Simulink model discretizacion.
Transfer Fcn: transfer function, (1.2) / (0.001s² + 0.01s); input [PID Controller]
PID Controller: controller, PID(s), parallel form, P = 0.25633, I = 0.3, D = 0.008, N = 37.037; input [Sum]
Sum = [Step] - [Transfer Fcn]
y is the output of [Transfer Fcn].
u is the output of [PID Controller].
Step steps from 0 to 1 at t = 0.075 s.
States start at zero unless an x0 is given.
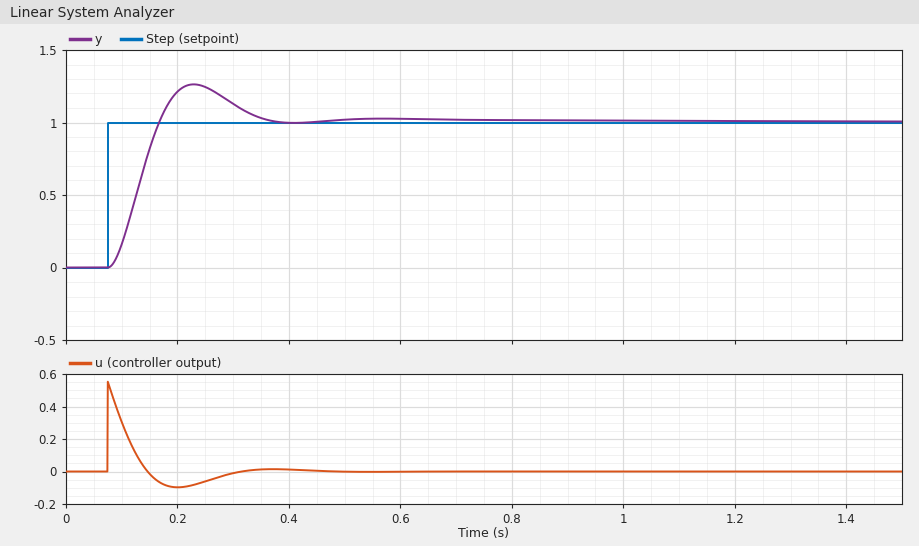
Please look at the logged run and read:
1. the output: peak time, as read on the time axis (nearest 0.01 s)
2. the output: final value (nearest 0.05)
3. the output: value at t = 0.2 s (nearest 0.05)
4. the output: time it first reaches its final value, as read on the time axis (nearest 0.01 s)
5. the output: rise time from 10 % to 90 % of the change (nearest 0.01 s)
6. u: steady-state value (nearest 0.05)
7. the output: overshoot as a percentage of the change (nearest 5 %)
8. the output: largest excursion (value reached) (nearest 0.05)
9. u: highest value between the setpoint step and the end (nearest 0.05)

0.23 s
1.00
1.20
0.17 s
0.06 s
0.00
25 %
1.25
0.55
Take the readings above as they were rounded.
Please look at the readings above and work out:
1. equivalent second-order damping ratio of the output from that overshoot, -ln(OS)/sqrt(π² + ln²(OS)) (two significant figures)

0.40
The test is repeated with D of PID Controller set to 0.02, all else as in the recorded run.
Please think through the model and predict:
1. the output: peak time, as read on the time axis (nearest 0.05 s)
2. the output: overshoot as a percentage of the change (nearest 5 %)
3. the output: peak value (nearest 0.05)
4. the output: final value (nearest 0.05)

0.20 s
15 %
1.15
1.00
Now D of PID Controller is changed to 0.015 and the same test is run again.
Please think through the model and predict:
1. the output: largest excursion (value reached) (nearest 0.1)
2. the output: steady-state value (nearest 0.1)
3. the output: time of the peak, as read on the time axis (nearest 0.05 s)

1.2
1.0
0.20 s
